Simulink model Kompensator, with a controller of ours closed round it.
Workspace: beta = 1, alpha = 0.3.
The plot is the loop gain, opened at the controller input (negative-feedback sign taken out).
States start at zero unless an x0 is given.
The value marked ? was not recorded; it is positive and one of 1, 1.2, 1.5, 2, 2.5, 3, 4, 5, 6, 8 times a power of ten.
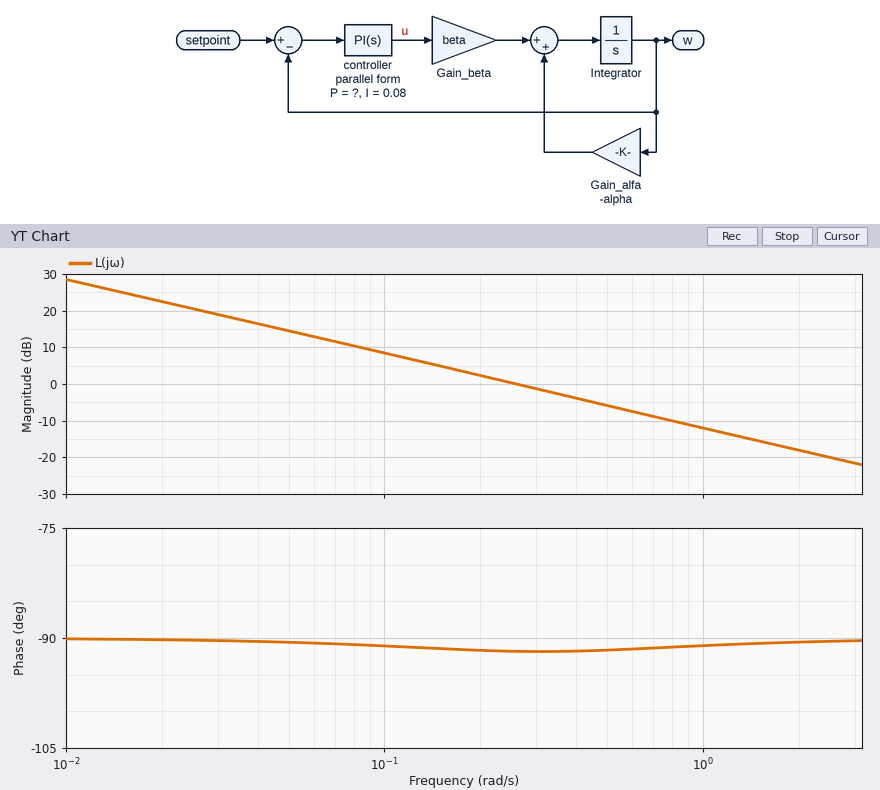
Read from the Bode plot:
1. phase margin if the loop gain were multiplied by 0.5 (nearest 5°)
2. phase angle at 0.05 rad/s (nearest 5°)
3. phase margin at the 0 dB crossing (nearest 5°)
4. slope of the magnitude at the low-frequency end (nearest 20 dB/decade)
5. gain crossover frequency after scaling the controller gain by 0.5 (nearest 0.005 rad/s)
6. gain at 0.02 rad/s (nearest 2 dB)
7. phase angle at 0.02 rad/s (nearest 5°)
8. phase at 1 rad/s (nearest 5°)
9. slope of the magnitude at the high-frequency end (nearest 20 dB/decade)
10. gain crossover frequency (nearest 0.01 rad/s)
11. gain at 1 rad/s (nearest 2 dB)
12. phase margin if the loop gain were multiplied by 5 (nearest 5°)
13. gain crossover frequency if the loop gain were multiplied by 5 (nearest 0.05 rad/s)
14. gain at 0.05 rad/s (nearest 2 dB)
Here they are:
90°
-90°
90°
-20 dB/decade
0.130 rad/s
22 dB
-90°
-90°
-20 dB/decade
0.26 rad/s
-12 dB
90°
1.25 rad/s
14 dB
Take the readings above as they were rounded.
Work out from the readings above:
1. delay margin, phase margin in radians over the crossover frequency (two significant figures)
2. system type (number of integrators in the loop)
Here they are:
6.0 s
1
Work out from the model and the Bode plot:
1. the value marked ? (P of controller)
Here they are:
0.25
